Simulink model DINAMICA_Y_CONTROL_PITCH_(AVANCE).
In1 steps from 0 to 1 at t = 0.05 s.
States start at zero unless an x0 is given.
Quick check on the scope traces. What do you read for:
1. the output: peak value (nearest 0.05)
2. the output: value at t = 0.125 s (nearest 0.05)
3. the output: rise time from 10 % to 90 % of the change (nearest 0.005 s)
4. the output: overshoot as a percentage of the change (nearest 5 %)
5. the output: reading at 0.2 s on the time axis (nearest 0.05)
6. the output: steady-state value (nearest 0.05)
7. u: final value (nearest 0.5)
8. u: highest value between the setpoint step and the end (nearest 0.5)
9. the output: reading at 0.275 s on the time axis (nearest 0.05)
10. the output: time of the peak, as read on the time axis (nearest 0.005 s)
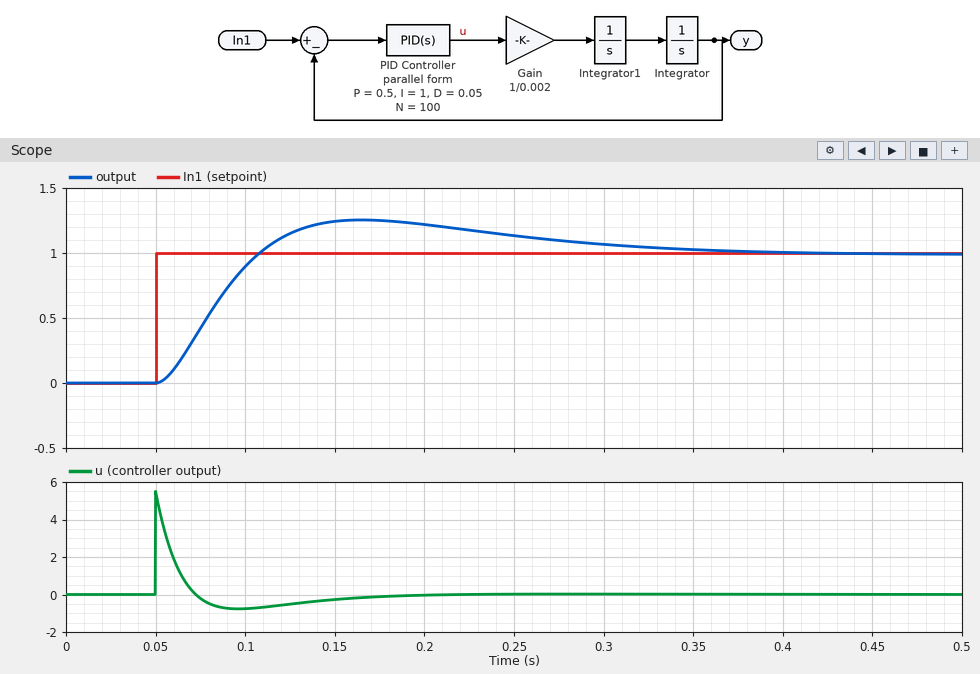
1.25
1.15
0.040 s
25 %
1.20
1.00
0.0
5.5
1.10
0.165 s
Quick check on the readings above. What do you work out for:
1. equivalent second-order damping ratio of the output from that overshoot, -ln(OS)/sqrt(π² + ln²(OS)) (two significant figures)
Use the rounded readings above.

0.40
